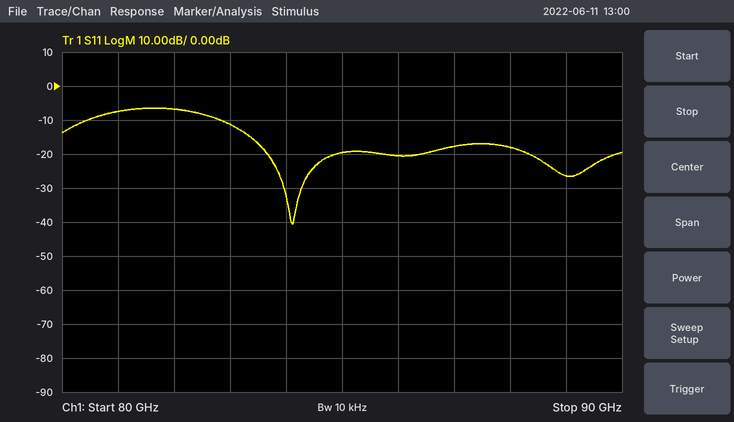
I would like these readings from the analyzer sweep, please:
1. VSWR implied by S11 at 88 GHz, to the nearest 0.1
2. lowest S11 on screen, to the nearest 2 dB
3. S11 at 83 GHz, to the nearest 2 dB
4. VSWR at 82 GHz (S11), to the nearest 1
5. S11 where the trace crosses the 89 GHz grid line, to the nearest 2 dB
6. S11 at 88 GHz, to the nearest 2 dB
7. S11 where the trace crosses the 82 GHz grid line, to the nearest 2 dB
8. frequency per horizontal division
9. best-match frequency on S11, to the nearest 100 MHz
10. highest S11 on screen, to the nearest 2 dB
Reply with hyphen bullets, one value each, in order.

- 1.3
- -40 dB
- -12 dB
- 3
- -26 dB
- -18 dB
- -6 dB
- 1 GHz
- 84.1 GHz
- -6 dB
